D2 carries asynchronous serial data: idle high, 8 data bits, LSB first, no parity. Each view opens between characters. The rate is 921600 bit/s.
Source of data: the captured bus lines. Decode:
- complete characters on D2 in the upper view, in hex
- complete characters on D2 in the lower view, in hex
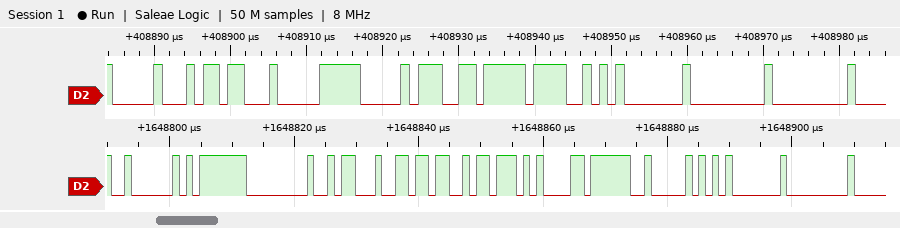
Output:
10, 1B, F0, D0, F6, 4F, 01, 00, 00
02, FD, 00, 1A, B6, DA, 85, 3F, 50, 01, 00
